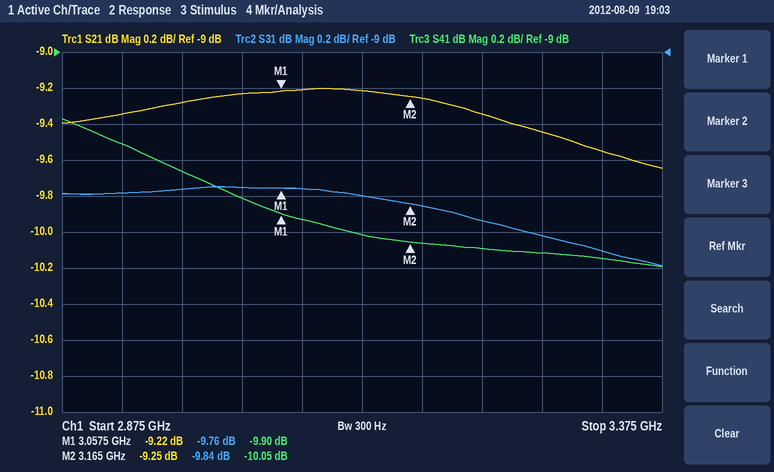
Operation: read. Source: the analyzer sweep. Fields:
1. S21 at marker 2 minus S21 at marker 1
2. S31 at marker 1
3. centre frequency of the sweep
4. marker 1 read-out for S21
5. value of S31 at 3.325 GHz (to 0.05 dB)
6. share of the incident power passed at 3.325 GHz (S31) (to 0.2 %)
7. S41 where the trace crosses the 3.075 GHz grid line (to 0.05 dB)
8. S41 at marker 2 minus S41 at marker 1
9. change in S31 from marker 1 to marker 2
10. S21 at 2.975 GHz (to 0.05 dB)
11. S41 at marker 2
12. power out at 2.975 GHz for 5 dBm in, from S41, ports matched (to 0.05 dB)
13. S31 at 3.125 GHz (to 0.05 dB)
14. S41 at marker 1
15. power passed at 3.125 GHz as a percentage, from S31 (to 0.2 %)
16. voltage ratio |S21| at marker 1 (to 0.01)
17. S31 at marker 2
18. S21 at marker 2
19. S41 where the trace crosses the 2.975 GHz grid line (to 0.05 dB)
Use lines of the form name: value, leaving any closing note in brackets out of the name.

S21 at marker 2 minus S21 at marker 1: -0.03 dB
S31 at marker 1: -9.76 dB
centre frequency of the sweep: 3.125 GHz
marker 1 read-out for S21: -9.22 dB
value of S31 at 3.325 GHz: -10.10 dB
share of the incident power passed at 3.325 GHz (S31): 9.8 %
S41 where the trace crosses the 3.075 GHz grid line: -9.95 dB
S41 at marker 2 minus S41 at marker 1: -0.15 dB
change in S31 from marker 1 to marker 2: -0.08 dB
S21 at 2.975 GHz: -9.30 dB
S41 at marker 2: -10.05 dB
power out at 2.975 GHz for 5 dBm in, from S41, ports matched: -4.65 dBm
S31 at 3.125 GHz: -9.80 dB
S41 at marker 1: -9.90 dB
power passed at 3.125 GHz as a percentage, from S31: 10.4 %
voltage ratio |S21| at marker 1: 0.35
S31 at marker 2: -9.84 dB
S21 at marker 2: -9.25 dB
S41 where the trace crosses the 2.975 GHz grid line: -9.65 dB
